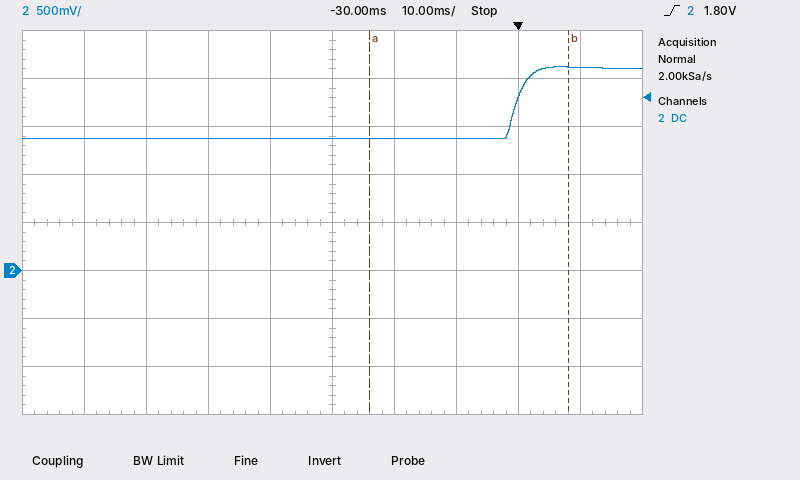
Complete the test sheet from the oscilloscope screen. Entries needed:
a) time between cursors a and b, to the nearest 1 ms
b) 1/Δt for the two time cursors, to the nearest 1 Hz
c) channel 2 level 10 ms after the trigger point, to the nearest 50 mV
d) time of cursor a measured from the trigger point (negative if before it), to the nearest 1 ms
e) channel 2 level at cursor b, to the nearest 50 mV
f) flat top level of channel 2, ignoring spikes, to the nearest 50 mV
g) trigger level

32 ms
31 Hz
2.10 V
-24 ms
2.10 V
2.10 V
1.80 V
